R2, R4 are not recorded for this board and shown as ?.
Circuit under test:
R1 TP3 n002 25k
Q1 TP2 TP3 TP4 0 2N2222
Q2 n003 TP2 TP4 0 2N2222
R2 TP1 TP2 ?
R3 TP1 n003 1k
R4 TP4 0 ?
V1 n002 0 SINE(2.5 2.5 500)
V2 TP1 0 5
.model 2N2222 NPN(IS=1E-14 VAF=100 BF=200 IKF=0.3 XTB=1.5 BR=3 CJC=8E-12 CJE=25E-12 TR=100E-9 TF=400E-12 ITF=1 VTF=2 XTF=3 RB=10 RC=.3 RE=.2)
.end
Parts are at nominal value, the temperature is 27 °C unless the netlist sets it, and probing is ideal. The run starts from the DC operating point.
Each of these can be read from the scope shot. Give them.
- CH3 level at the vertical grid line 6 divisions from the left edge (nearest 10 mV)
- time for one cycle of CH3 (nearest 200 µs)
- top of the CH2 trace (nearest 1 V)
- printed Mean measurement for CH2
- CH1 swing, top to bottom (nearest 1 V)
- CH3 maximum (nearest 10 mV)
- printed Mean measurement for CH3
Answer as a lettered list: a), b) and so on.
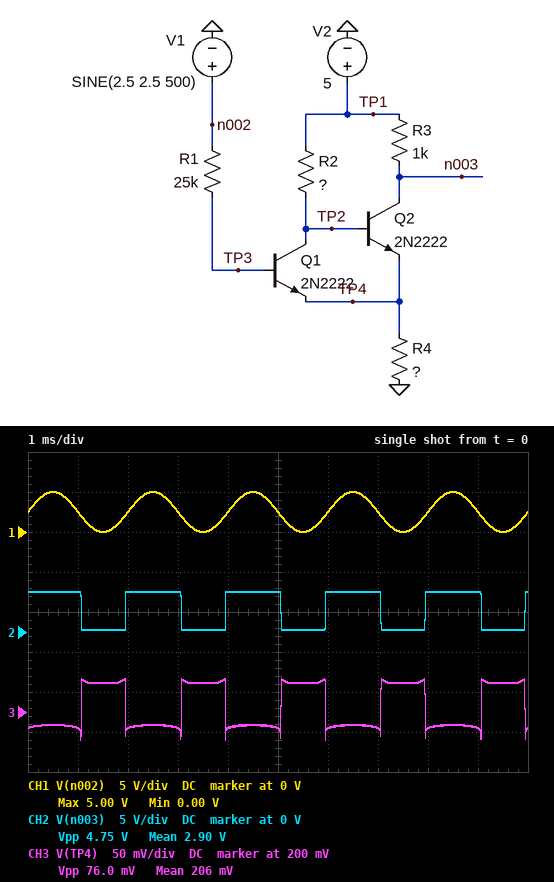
a) 180 mV
b) 2.0 ms
c) 5 V
d) 2.90 V
e) 5 V
f) 240 mV
g) 206 mV
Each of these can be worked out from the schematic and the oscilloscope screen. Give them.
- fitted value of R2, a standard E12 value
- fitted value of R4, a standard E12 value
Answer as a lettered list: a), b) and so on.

a) 470 Ω
b) 18 Ω
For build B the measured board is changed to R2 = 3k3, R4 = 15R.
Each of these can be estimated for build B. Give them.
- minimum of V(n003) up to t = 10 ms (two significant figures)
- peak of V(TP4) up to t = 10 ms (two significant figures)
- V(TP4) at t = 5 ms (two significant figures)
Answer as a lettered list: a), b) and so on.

a) 120 mV
b) 92 mV
c) 23 mV
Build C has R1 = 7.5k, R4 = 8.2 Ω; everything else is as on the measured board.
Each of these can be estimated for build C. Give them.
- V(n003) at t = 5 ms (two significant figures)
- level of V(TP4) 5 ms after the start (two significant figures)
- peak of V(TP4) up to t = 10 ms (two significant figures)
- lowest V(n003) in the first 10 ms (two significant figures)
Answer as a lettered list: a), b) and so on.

a) 5.0 V
b) 86 mV
c) 110 mV
d) 130 mV
